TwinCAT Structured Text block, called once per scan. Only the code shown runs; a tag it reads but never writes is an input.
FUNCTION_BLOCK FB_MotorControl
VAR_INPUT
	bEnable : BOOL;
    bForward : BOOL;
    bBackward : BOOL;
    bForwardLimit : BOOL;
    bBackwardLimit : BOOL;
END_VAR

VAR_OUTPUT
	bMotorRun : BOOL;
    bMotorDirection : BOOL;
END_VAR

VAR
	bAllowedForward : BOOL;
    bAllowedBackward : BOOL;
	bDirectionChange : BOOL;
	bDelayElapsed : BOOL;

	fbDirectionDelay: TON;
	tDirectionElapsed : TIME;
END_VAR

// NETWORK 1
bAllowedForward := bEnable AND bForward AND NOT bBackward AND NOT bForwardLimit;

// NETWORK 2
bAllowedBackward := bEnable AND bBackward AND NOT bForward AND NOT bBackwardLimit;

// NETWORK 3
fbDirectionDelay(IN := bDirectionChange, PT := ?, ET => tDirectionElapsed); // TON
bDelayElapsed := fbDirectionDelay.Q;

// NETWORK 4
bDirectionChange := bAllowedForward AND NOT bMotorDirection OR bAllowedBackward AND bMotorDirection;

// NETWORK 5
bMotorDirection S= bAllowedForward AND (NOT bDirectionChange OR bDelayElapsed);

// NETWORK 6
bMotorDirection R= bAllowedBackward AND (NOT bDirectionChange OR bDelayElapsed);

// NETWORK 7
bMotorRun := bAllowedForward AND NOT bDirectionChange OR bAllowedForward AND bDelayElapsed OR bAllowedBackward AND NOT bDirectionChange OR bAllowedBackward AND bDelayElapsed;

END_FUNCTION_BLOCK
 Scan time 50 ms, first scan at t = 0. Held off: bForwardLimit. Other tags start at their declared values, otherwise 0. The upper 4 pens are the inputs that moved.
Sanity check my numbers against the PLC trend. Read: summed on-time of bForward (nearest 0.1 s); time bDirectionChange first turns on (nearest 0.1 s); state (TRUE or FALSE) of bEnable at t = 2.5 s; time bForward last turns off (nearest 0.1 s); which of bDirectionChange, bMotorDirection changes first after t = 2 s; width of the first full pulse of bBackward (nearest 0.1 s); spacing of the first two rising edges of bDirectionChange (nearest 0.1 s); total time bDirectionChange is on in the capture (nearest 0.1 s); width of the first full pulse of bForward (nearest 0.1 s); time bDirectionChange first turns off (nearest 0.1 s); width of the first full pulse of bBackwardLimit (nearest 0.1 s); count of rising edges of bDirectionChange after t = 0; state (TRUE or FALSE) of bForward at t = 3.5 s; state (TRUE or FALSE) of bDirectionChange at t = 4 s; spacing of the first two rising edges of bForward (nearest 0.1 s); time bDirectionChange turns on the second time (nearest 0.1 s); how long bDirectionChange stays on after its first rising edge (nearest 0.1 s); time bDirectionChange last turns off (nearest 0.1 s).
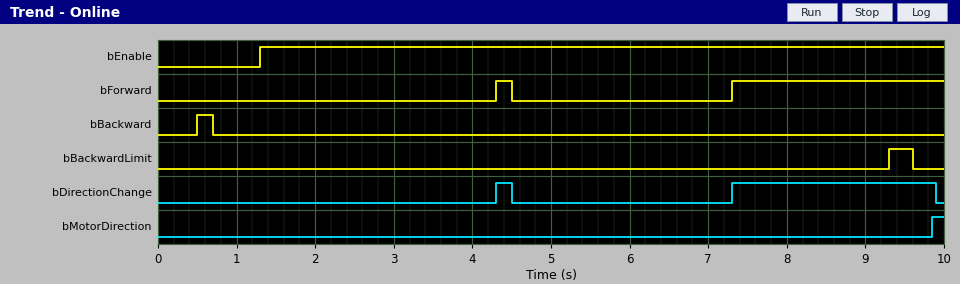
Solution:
2.9 s
4.3 s
TRUE
4.5 s
bDirectionChange
0.2 s
3.0 s
2.8 s
0.2 s
4.5 s
0.3 s
2
FALSE
FALSE
3.0 s
7.3 s
0.2 s
9.9 s
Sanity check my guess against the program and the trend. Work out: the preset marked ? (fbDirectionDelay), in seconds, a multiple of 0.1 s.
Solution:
2.5 s
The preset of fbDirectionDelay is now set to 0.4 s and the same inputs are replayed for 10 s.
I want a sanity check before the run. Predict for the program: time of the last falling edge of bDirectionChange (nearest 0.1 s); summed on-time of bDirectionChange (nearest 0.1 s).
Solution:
7.8 s
0.7 s
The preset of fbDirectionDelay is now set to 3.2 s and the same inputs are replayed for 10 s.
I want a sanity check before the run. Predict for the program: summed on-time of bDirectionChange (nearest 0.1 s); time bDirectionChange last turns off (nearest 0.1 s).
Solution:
2.9 s
4.5 s
